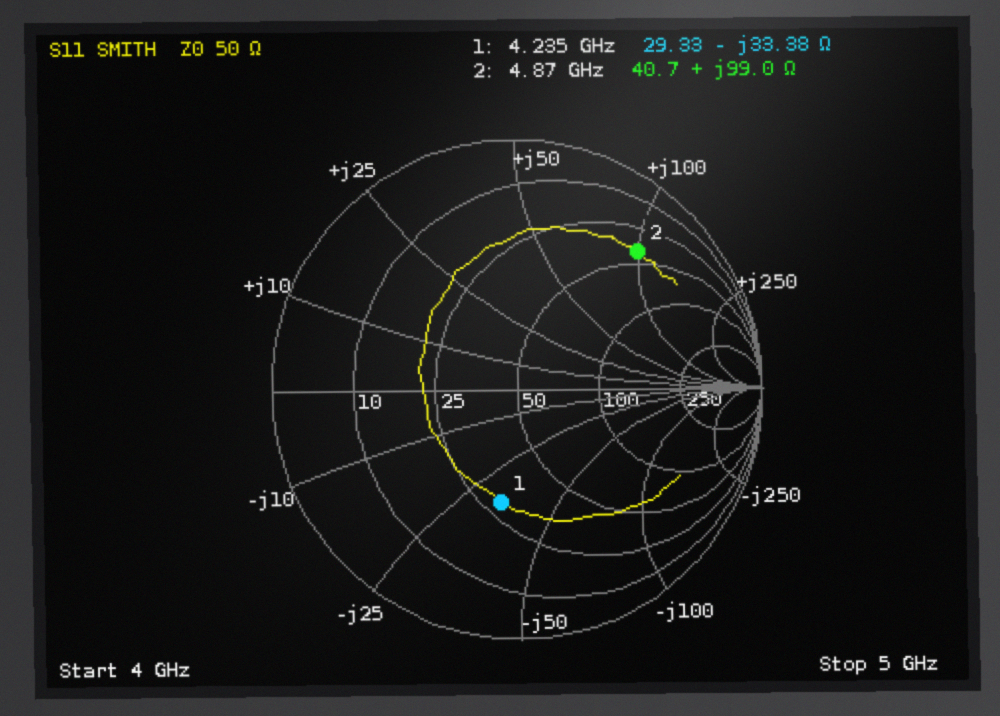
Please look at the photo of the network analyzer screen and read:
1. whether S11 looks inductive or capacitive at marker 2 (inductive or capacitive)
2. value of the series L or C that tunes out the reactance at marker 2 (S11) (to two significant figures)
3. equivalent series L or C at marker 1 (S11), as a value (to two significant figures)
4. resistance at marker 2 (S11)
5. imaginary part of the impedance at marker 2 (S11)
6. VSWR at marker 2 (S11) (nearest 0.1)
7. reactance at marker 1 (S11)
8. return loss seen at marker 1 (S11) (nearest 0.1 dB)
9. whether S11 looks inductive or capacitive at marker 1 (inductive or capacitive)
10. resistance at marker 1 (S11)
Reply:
inductive
330 fF
1.1 pF
40.7 Ω
+99.0 Ω
6.7
-33.38 Ω
6.8 dB
capacitive
29.33 Ω
